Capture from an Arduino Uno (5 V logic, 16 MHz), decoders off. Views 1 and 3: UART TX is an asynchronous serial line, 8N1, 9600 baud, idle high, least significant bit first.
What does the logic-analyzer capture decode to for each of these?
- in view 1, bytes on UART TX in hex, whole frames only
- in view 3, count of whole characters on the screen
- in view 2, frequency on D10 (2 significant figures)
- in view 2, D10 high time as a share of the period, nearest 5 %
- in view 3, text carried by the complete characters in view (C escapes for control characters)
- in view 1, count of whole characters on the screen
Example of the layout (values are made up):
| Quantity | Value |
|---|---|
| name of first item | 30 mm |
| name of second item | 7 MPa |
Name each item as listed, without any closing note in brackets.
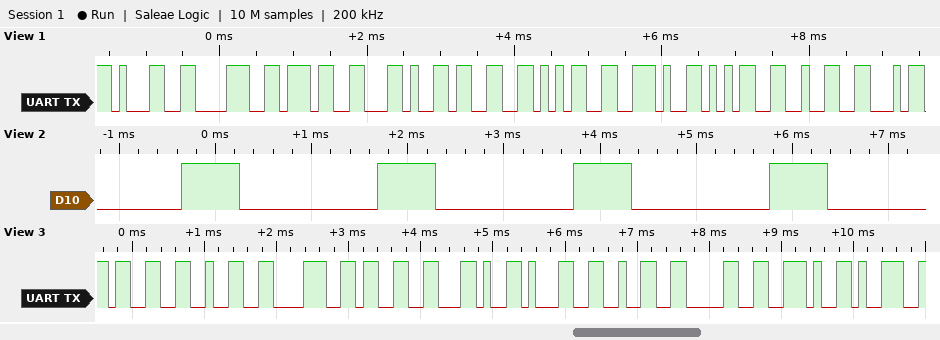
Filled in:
| Quantity | Value |
|---|---|
| in view 1, bytes on UART TX in hex, whole frames only | 31 38 37 2C 33 35 2E 35 32 |
| in view 3, count of whole characters on the screen | 10 |
| in view 2, frequency on D10 | 490 Hz |
| in view 2, D10 high time as a share of the period, nearest 5 % | 30 % |
| in view 3, text carried by the complete characters in view | "3283,120.9" |
| in view 1, count of whole characters on the screen | 9 |
